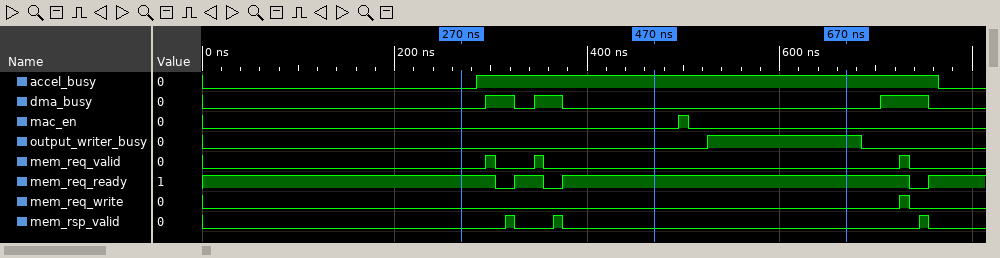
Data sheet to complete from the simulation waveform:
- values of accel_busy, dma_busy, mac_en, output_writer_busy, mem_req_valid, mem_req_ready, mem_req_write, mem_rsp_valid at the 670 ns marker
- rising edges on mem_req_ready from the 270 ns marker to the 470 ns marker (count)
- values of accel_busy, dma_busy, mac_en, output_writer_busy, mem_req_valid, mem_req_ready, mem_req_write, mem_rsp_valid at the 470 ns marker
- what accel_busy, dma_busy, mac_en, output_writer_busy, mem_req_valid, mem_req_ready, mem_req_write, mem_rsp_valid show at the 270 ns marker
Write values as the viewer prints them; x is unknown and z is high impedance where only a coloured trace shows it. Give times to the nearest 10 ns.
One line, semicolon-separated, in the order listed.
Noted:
accel_busy=1, dma_busy=0, mac_en=0, output_writer_busy=1, mem_req_valid=0, mem_req_ready=1, mem_req_write=0, mem_rsp_valid=0; 2; accel_busy=1, dma_busy=0, mac_en=0, output_writer_busy=0, mem_req_valid=0, mem_req_ready=1, mem_req_write=0, mem_rsp_valid=0; accel_busy=0, dma_busy=0, mac_en=0, output_writer_busy=0, mem_req_valid=0, mem_req_ready=1, mem_req_write=0, mem_rsp_valid=0
